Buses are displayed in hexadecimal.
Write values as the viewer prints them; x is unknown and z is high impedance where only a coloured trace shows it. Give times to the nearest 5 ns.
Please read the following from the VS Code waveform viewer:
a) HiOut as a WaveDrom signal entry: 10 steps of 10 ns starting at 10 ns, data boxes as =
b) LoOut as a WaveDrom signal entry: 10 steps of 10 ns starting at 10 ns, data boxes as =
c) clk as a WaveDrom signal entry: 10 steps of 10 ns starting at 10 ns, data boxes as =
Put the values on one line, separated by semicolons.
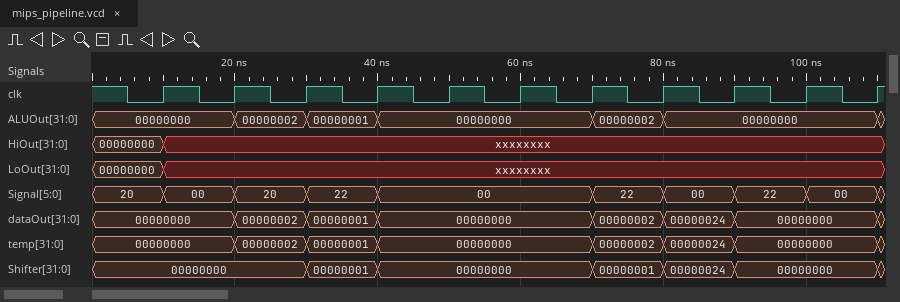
{name: 'HiOut', wave: 'x.........'}; {name: 'LoOut', wave: 'x.........'}; {name: 'clk', wave: 'p.........'}
